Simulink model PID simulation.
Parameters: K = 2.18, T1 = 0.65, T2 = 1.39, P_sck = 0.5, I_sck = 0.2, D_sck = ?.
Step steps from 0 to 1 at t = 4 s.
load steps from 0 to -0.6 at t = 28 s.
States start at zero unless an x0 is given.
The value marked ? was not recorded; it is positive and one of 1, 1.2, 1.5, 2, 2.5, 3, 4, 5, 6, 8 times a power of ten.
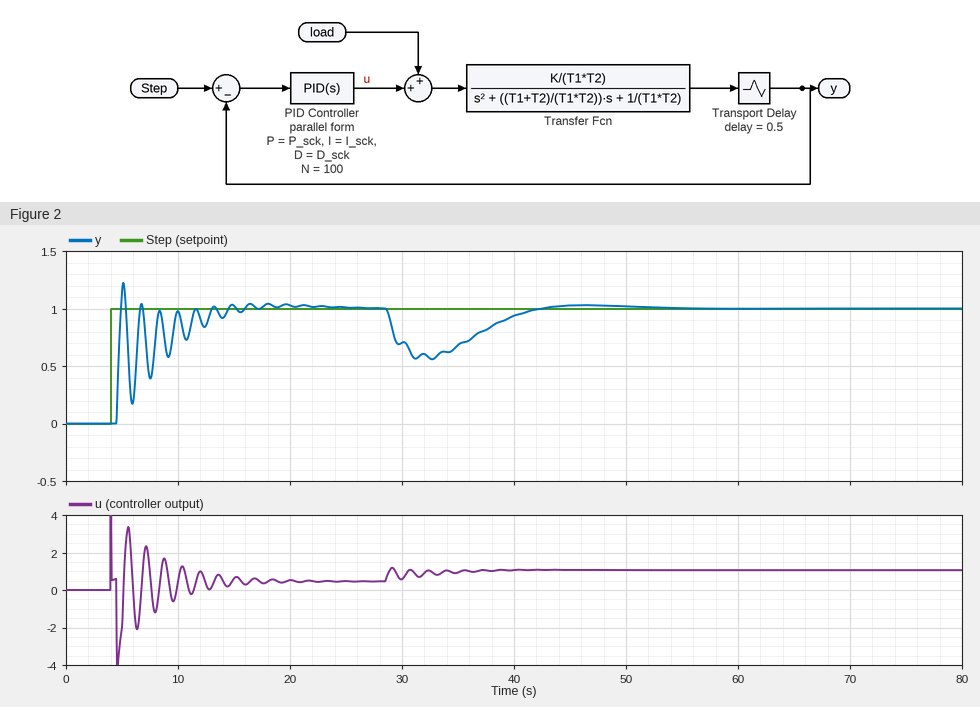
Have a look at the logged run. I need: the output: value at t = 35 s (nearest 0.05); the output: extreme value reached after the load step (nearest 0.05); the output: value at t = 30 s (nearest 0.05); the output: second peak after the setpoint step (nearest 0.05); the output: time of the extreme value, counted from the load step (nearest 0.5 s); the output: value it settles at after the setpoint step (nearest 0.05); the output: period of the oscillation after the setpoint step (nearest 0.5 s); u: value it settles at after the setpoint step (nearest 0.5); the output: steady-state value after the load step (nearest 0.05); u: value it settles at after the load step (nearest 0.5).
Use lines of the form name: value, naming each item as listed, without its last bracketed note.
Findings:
the output: value at t = 35 s: 0.70
the output: extreme value reached after the load step: 0.55
the output: value at t = 30 s: 0.70
the output: second peak after the setpoint step: 1.05
the output: time of the extreme value, counted from the load step: 4.5 s
the output: value it settles at after the setpoint step: 1.00
the output: period of the oscillation after the setpoint step: 1.5 s
u: value it settles at after the setpoint step: 0.5
the output: steady-state value after the load step: 1.00
u: value it settles at after the load step: 1.0
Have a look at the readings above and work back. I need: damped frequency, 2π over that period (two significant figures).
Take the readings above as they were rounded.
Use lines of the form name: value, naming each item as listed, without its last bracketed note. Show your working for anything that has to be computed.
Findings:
damped frequency, 2π over that period: 2π / 1.5 = 4.2 rad/s
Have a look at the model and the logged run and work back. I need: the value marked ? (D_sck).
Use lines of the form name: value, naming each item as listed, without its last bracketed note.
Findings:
the value marked ?: 1.5
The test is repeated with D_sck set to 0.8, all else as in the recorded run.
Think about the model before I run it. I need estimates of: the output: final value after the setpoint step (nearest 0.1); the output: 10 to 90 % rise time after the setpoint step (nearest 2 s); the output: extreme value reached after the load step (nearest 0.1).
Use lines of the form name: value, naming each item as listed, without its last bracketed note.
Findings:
the output: final value after the setpoint step: 1.0
the output: 10 to 90 % rise time after the setpoint step: 6 s
the output: extreme value reached after the load step: 0.5
